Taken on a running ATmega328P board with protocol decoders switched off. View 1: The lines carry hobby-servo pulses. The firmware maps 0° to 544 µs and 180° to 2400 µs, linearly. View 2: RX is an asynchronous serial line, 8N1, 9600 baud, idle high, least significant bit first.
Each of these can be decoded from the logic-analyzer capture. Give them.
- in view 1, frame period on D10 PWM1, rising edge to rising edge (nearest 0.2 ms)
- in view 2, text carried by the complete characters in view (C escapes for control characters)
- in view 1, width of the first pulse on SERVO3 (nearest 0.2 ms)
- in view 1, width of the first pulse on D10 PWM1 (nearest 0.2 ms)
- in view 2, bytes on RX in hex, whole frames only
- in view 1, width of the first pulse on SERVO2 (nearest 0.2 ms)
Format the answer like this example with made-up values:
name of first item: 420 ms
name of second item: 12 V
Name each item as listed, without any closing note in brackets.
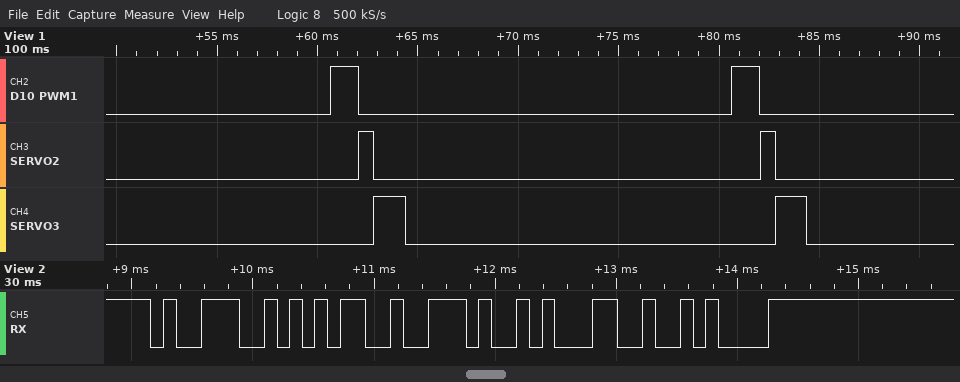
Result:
in view 1, frame period on D10 PWM1, rising edge to rising edge: 20.0 ms
in view 2, text carried by the complete characters in view: "95.1\n"
in view 1, width of the first pulse on SERVO3: 1.6 ms
in view 1, width of the first pulse on D10 PWM1: 1.4 ms
in view 2, bytes on RX in hex, whole frames only: 39 35 2E 31 0A
in view 1, width of the first pulse on SERVO2: 0.8 ms
